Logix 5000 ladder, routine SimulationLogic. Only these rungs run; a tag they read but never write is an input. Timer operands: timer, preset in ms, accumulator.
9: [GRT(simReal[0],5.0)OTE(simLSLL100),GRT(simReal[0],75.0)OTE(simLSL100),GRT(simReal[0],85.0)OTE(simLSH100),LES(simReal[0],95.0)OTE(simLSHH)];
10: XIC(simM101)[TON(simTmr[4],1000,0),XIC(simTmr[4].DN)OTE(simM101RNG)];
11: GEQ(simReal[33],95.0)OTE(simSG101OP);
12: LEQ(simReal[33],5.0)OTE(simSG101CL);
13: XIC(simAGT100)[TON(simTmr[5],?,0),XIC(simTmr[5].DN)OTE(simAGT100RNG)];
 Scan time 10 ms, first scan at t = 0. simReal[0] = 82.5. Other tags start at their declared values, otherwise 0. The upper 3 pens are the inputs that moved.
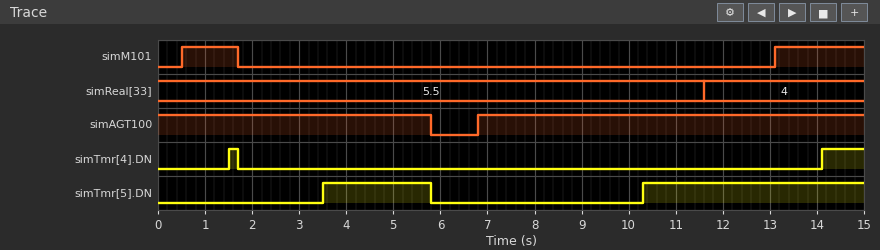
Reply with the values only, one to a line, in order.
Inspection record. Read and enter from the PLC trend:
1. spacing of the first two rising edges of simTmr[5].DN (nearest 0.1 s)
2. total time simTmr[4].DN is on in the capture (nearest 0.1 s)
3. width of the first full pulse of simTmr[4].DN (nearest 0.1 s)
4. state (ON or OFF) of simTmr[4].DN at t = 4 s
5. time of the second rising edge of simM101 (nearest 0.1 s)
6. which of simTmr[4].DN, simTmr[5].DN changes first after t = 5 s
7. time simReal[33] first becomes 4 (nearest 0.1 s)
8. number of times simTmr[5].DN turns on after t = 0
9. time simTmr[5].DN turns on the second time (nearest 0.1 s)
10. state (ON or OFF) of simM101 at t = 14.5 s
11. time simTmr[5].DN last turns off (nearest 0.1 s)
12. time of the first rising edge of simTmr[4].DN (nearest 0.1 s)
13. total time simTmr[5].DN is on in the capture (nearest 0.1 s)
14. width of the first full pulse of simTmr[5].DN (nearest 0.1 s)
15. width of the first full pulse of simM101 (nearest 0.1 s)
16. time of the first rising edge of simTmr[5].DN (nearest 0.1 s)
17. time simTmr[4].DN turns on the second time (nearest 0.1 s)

6.8 s
1.1 s
0.2 s
OFF
13.1 s
simTmr[5].DN
11.6 s
2
10.3 s
ON
5.8 s
1.5 s
7.0 s
2.3 s
1.2 s
3.5 s
14.1 s
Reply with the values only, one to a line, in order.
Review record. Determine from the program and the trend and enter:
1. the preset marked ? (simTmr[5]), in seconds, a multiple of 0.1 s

3.5 s
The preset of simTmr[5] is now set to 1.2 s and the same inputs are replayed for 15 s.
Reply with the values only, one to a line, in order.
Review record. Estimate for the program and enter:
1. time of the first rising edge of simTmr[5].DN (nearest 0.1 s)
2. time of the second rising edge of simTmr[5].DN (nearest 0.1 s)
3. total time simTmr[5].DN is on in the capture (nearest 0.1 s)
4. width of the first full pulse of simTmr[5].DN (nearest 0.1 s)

1.2 s
8.0 s
11.6 s
4.6 s
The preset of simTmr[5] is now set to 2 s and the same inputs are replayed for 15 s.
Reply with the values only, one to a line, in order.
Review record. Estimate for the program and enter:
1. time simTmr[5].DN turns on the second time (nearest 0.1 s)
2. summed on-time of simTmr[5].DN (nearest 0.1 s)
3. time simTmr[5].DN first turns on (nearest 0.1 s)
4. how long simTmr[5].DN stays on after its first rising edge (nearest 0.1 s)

8.8 s
10.0 s
2.0 s
3.8 s
